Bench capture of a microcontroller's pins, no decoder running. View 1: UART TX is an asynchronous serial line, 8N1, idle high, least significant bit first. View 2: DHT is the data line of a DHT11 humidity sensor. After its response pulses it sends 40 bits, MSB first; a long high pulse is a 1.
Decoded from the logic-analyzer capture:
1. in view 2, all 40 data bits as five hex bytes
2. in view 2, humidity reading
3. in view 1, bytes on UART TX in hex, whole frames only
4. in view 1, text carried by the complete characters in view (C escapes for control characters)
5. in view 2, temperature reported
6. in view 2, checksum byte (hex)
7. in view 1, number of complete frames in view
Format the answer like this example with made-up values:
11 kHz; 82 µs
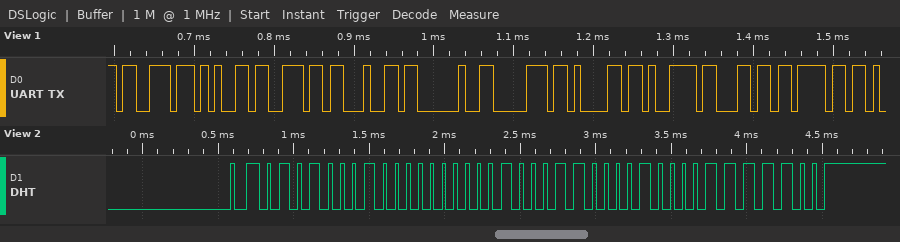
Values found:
51 00 23 08 7C; 81 %; 0x73 0x65 0x6E 0x64 0x20 0x70 0x61 0x79 0x6C 0x6F; "send paylo"; 35.8 °C; 0x7C; 10
